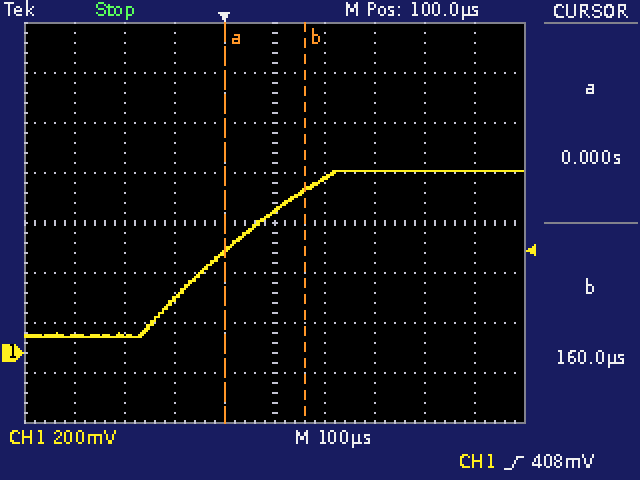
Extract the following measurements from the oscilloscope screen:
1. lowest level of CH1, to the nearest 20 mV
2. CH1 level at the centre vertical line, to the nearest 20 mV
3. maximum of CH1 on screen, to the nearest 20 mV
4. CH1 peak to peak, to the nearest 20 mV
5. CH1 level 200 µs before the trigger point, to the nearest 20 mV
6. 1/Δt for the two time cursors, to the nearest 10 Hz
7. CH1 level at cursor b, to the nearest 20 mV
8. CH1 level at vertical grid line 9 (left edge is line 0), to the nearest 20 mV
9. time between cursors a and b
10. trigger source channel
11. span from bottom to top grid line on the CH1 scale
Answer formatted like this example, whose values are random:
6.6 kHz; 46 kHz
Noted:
60 mV; 560 mV; 720 mV; 660 mV; 60 mV; 6.25 kHz; 660 mV; 720 mV; 160 µs; CH1; 1.6 V
